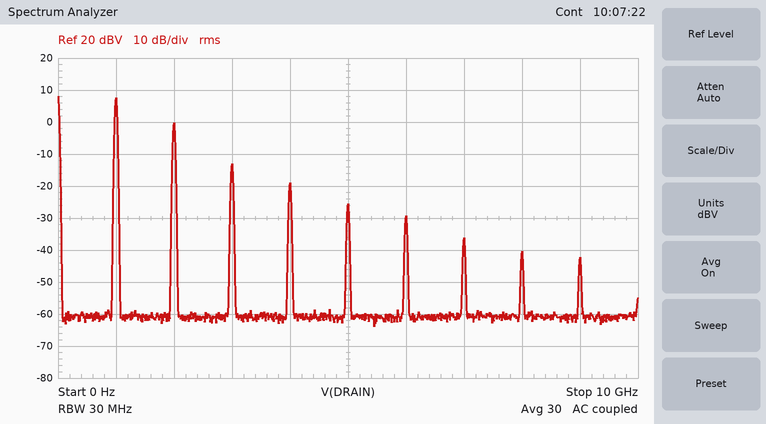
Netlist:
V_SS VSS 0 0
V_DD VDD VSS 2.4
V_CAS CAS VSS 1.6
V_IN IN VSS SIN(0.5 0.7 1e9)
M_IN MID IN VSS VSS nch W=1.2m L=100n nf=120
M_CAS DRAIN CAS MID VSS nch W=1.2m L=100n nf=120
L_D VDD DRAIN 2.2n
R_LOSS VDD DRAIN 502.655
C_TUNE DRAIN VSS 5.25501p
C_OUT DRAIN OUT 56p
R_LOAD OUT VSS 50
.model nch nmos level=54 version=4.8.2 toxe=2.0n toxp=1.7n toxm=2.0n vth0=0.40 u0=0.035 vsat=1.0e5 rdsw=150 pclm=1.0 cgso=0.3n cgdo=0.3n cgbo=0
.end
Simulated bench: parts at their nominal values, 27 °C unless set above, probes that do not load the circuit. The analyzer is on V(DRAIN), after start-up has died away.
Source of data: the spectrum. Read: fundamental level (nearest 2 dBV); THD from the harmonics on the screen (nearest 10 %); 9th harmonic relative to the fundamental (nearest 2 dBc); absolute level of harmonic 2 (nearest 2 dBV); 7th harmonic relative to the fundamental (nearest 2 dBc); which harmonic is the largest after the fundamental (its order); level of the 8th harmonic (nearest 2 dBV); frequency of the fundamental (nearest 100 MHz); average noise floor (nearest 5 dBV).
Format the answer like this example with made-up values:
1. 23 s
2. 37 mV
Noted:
1. 8 dBV
2. 40 %
3. -50 dBc
4. 0 dBV
5. -44 dBc
6. 2
7. -40 dBV
8. 1.0 GHz
9. -60 dBV
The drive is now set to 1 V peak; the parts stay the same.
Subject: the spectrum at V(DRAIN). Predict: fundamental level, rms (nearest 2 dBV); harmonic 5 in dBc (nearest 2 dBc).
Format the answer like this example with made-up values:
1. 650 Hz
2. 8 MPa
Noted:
1. 8 dBV
2. -30 dBc
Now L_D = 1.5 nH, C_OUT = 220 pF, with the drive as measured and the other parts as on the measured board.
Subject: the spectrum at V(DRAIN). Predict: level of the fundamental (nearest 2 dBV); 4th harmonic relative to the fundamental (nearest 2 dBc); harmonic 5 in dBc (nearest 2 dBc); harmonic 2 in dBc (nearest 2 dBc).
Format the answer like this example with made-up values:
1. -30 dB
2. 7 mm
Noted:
1. 8 dBV
2. -24 dBc
3. -32 dBc
4. -4 dBc
